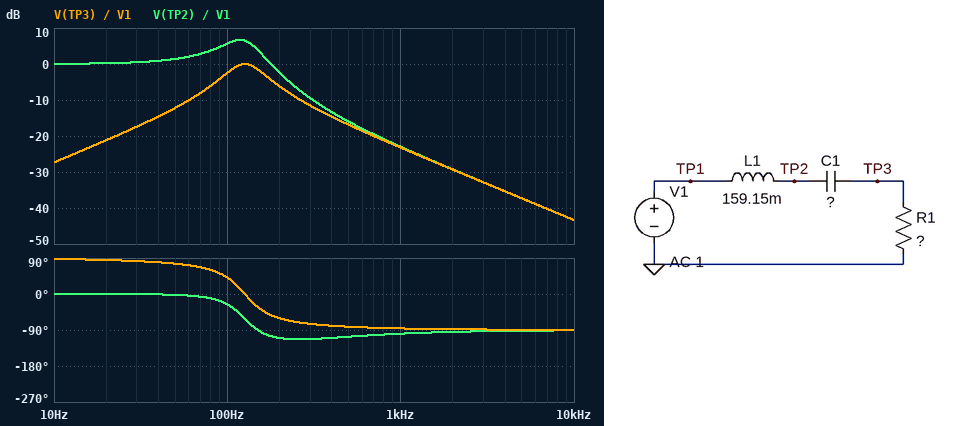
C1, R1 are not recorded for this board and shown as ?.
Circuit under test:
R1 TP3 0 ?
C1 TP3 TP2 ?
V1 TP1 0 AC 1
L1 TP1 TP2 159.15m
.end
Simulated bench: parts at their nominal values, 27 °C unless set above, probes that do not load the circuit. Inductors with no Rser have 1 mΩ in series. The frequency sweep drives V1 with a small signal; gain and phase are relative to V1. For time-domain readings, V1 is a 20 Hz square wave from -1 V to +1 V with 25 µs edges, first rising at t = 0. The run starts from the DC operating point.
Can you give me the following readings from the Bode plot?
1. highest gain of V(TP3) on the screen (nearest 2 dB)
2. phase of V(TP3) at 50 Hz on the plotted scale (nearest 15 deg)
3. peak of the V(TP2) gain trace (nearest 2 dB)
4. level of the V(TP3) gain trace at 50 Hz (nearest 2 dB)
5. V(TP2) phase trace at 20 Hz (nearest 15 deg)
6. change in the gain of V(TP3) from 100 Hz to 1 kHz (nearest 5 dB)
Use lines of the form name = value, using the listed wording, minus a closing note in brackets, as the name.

highest gain of V(TP3) on the screen = 0 dB
phase of V(TP3) at 50 Hz on the plotted scale = 75 deg
peak of the V(TP2) gain trace = 6 dB
level of the V(TP3) gain trace at 50 Hz = -12 dB
V(TP2) phase trace at 20 Hz = 0 deg
change in the gain of V(TP3) from 100 Hz to 1 kHz = -20 dB
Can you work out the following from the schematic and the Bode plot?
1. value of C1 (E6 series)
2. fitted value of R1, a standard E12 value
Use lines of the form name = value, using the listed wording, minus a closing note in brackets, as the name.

value of C1 = 10 µF
fitted value of R1, a standard E12 value = 68 Ω
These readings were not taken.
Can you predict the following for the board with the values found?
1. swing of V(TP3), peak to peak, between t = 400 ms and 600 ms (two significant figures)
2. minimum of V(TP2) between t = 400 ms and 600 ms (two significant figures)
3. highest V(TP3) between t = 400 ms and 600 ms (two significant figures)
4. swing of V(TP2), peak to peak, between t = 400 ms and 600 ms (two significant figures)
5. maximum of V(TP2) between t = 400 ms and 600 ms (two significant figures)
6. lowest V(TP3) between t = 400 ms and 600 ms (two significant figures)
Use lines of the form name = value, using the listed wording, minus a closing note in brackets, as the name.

swing of V(TP3), peak to peak, between t = 400 ms and 600 ms = 1.5 V
minimum of V(TP2) between t = 400 ms and 600 ms = -2.0 V
highest V(TP3) between t = 400 ms and 600 ms = 750 mV
swing of V(TP2), peak to peak, between t = 400 ms and 600 ms = 3.9 V
maximum of V(TP2) between t = 400 ms and 600 ms = 2.0 V
lowest V(TP3) between t = 400 ms and 600 ms = -750 mV
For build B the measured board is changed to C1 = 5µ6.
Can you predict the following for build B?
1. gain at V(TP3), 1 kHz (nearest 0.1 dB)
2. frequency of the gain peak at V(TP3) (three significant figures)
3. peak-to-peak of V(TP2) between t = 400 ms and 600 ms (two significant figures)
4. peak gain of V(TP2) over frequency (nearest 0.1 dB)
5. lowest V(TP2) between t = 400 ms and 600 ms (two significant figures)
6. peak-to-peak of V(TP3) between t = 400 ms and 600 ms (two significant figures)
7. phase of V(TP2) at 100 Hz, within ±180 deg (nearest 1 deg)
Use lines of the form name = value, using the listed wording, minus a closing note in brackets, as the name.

gain at V(TP3), 1 kHz = -23.1 dB
frequency of the gain peak at V(TP3) = 169 Hz
peak-to-peak of V(TP2) between t = 400 ms and 600 ms = 4.3 V
peak gain of V(TP2) over frequency = 8.7 dB
lowest V(TP2) between t = 400 ms and 600 ms = -2.1 V
peak-to-peak of V(TP3) between t = 400 ms and 600 ms = 1.2 V
phase of V(TP2) at 100 Hz, within ±180 deg = -7 deg
